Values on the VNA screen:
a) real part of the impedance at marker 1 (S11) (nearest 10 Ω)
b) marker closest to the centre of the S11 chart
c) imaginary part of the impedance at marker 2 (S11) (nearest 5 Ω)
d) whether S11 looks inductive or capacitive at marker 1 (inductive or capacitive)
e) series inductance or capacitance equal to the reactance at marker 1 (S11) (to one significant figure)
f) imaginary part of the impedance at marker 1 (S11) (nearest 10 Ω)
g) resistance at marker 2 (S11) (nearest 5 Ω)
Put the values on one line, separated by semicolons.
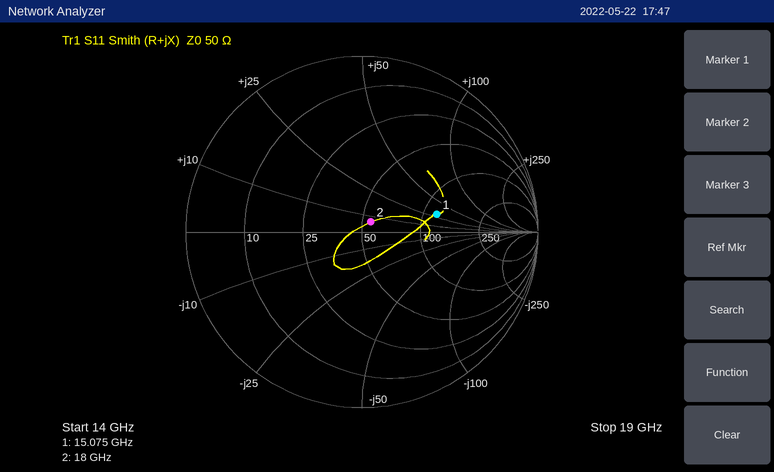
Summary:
120 Ω; marker 2; +5 Ω; inductive; 300 pH; +30 Ω; 55 Ω
